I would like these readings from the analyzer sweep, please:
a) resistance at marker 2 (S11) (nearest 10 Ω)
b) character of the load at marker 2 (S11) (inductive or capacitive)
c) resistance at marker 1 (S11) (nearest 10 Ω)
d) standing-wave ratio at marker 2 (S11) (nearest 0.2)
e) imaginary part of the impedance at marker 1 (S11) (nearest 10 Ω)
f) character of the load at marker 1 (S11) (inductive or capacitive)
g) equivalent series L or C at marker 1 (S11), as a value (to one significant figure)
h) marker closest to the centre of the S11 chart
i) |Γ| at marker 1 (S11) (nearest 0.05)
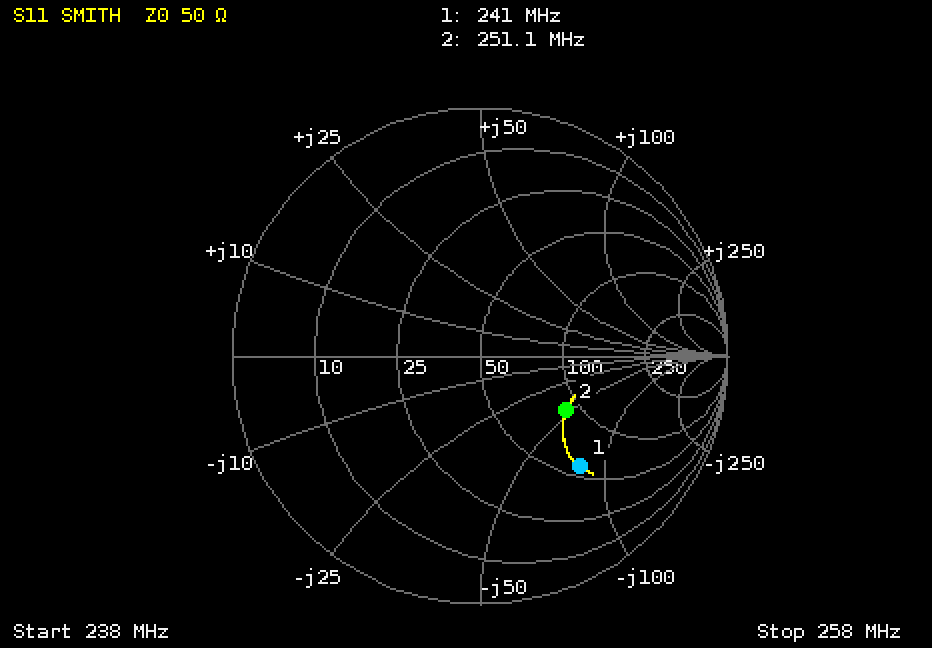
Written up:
90 Ω
capacitive
60 Ω
2.4
-80 Ω
capacitive
8 pF
marker 2
0.60
